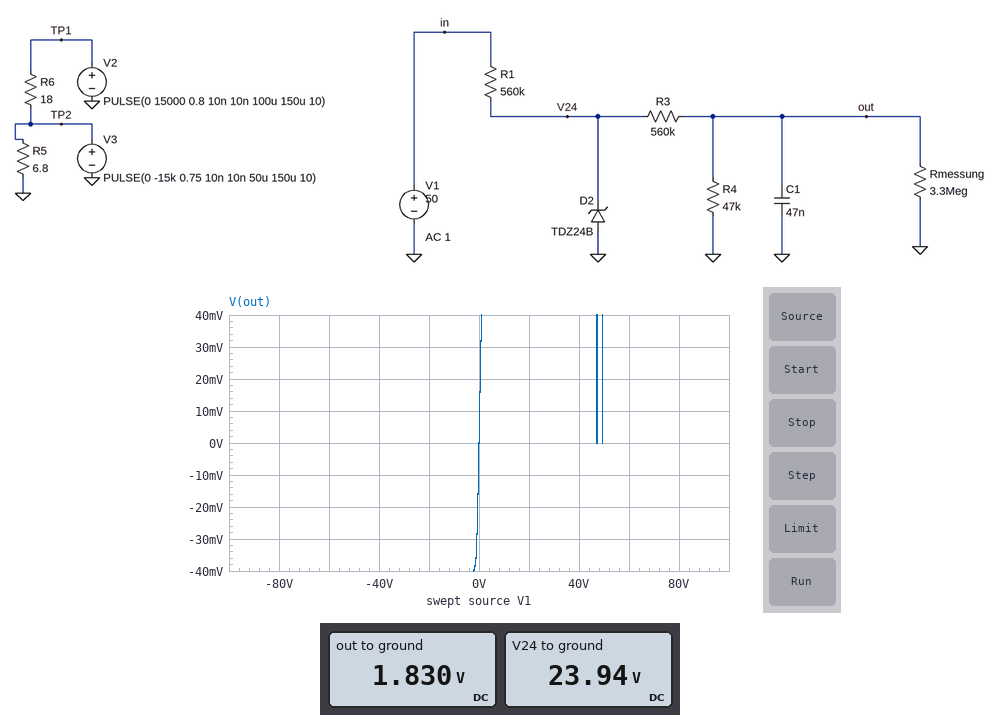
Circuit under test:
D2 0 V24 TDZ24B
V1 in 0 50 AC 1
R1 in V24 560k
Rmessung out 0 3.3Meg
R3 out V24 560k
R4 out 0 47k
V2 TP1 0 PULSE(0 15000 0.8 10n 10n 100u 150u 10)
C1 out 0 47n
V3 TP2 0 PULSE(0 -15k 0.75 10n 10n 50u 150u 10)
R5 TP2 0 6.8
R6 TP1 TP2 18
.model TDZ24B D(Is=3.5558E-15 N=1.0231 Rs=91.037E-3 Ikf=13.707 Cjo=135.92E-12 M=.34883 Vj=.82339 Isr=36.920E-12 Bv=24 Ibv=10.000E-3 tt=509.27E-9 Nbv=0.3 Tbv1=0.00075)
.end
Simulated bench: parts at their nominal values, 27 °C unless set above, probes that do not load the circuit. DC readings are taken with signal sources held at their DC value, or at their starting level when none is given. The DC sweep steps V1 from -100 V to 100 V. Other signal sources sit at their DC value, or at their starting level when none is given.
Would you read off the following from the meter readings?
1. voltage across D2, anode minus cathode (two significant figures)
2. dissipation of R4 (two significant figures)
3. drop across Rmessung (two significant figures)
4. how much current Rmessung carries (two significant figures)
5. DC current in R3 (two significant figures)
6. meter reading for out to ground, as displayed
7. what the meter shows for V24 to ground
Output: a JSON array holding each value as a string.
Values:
["-24 V", "71 µW", "1.8 V", "550 nA", "39 µA", "1.830 V", "23.94 V"]
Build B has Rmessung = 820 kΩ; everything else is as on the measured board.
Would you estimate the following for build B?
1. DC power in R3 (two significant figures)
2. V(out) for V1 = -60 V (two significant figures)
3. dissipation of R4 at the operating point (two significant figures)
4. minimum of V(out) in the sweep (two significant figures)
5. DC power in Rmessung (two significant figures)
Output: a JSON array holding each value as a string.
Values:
["880 µW", "-47 mV", "66 µW", "-48 mV", "3.8 µW"]
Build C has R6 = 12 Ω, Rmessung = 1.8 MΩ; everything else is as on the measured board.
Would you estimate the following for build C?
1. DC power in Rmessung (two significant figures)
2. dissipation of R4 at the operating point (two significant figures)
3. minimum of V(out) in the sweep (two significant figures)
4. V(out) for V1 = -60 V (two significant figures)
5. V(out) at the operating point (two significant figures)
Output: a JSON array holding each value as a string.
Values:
["1.8 µW", "70 µW", "-49 mV", "-48 mV", "1.8 V"]
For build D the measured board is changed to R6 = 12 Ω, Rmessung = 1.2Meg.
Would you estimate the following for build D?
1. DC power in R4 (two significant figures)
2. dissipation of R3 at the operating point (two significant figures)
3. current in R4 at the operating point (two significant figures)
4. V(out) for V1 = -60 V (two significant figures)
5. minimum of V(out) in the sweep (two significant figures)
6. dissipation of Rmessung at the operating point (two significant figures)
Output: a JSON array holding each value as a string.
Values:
["68 µW", "880 µW", "38 µA", "-48 mV", "-49 mV", "2.7 µW"]
